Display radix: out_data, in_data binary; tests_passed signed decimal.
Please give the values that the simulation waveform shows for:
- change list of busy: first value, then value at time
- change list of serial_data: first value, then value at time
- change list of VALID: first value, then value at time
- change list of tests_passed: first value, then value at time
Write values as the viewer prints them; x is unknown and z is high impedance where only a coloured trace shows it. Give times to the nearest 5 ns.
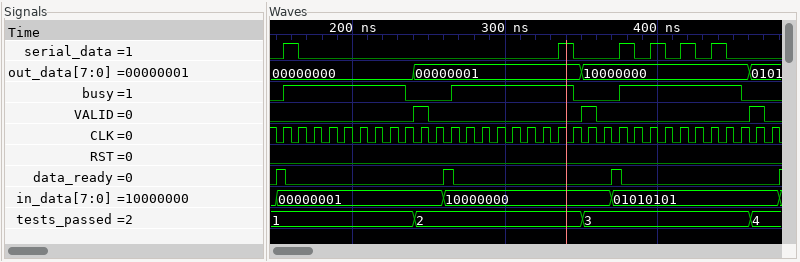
0, 1 at 155 ns, 0 at 235 ns, 1 at 265 ns, 0 at 345 ns, 1 at 375 ns, 0 at 455 ns
0, 1 at 155 ns, 0 at 165 ns, 1 at 335 ns, 0 at 345 ns, 1 at 375 ns, 0 at 385 ns, 1 at 395 ns, 0 at 405 ns, 1 at 415 ns, 0 at 425 ns, 1 at 435 ns, 0 at 445 ns
0, 1 at 240 ns, 0 at 250 ns, 1 at 350 ns, 0 at 360 ns, 1 at 460 ns, 0 at 470 ns
1, 2 at 240 ns, 3 at 350 ns, 4 at 460 ns
